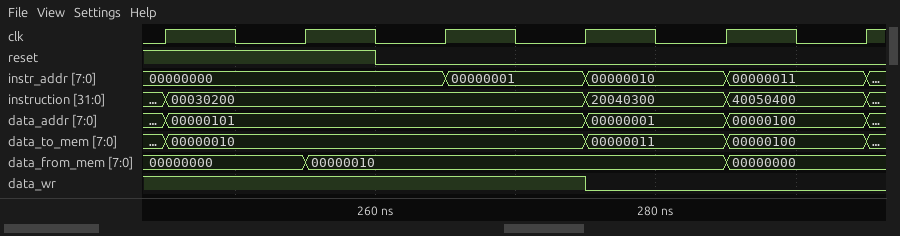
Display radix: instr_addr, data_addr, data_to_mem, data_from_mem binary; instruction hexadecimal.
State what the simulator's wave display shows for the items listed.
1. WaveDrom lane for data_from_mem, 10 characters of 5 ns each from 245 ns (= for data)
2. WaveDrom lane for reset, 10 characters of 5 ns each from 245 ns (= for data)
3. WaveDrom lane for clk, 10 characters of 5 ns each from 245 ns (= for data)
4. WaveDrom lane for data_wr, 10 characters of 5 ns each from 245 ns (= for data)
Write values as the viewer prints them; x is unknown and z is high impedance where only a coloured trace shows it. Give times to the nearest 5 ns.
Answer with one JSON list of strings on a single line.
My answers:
["{name: 'data_from_mem', wave: '=.=.....=.', data: '00000000 00000010 00000000'}", "{name: 'reset', wave: '1..0......'}", "{name: 'clk', wave: '1010101010'}", "{name: 'data_wr', wave: '1.....0...'}"]
